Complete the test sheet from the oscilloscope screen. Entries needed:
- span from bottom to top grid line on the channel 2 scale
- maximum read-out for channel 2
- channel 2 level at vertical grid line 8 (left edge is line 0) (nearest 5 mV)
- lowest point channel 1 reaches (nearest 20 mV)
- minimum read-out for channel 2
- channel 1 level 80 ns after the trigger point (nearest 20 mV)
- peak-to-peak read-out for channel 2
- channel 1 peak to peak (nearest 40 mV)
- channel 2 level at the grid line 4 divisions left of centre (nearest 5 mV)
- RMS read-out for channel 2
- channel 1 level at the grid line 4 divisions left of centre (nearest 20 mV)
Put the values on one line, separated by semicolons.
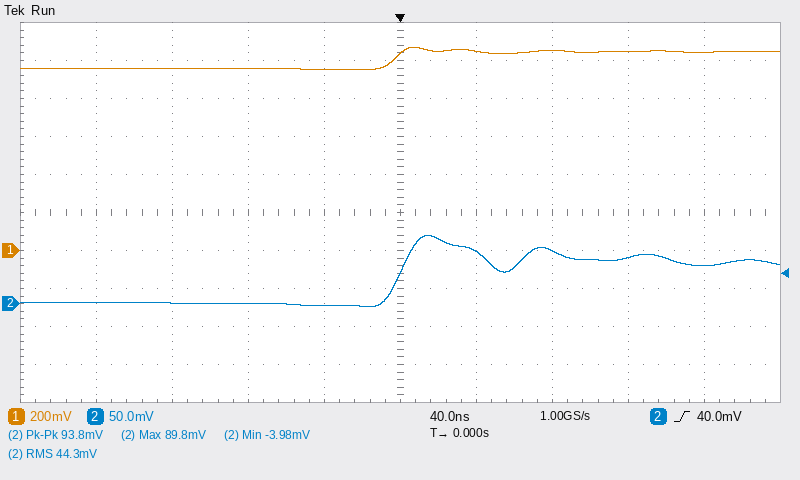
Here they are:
500 mV; 89.8 mV; 60 mV; 960 mV; -3.98 mV; 1.06 V; 93.8 mV; 120 mV; 0 mV; 44.3 mV; 960 mV
